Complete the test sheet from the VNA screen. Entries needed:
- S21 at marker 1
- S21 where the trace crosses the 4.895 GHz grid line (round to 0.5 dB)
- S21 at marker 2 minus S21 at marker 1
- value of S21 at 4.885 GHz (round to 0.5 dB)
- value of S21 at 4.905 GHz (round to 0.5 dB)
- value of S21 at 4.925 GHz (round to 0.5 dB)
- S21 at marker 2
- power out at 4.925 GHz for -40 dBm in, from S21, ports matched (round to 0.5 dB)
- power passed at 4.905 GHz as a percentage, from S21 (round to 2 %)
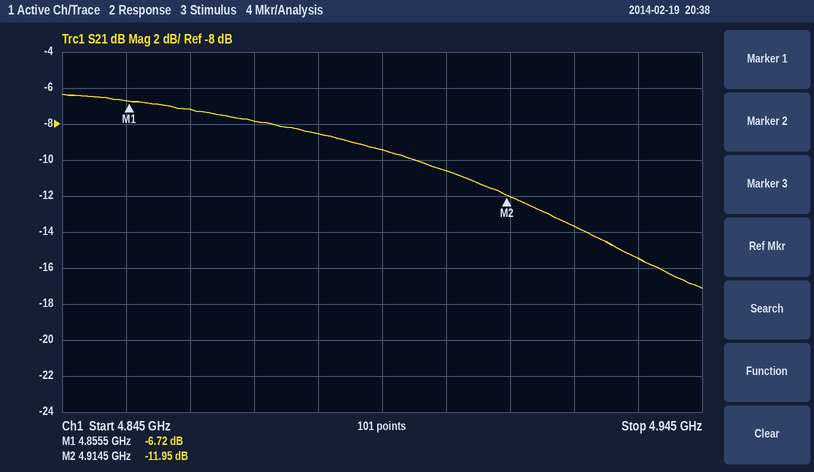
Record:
-6.72 dB
-9.5 dB
-5.23 dB
-8.5 dB
-10.5 dB
-13.5 dB
-11.95 dB
-53.5 dBm
8 %
